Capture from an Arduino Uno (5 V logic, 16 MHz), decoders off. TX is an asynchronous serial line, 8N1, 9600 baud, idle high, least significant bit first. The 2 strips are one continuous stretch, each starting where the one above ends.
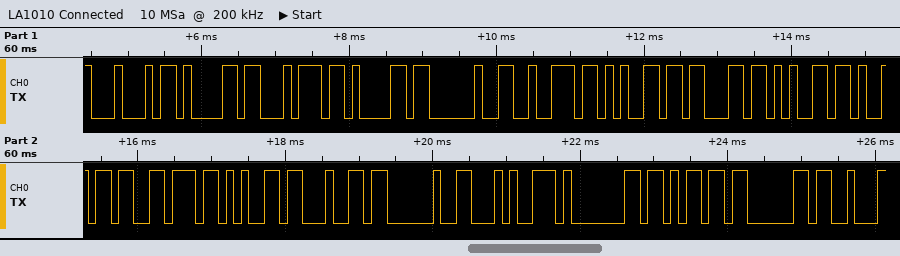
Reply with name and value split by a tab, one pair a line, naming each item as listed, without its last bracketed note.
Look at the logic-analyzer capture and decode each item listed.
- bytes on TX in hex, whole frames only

bytes on TX in hex, whole frames only	0x44 0x61 0x74 0x61 0x20 0x72 0x65 0x63 0x65 0x69 0x76 0x65 0x64 0x20 0x94 0x01 0x6B 0x03 0x13
